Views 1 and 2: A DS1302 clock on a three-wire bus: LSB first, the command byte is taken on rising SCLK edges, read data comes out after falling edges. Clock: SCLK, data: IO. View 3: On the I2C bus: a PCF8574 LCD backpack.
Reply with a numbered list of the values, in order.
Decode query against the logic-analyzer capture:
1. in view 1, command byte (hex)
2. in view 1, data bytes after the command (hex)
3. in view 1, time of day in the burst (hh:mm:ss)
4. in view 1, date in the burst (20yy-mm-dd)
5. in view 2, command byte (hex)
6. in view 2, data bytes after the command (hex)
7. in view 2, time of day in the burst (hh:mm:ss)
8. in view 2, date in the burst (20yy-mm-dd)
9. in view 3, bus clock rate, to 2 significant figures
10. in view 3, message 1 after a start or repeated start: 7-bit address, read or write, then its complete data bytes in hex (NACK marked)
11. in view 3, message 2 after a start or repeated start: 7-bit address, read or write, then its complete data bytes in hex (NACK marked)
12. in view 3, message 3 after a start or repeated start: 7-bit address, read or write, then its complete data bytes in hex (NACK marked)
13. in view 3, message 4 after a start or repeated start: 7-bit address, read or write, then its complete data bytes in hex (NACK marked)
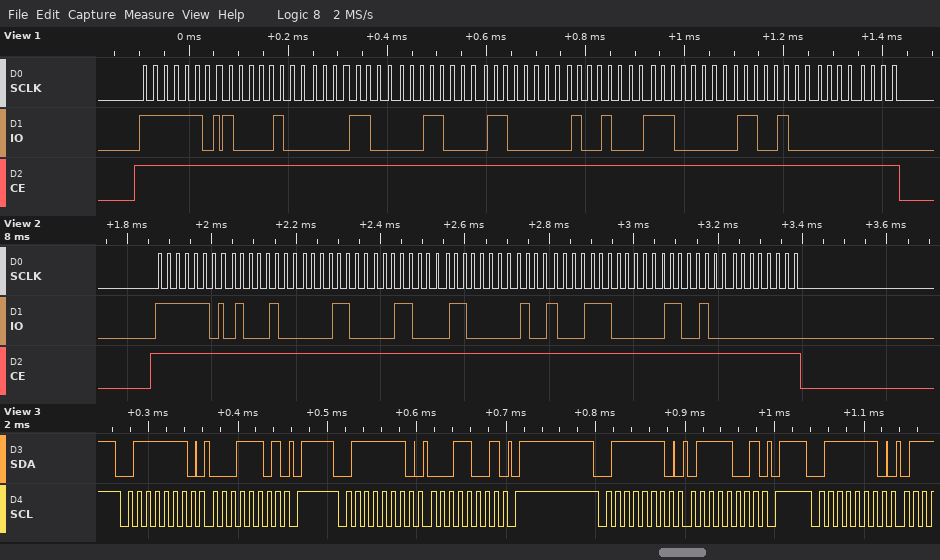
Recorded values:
1. 0xBF
2. 21 30 18 06 12 07 26 00
3. 18:30:21
4. 2026-12-06
5. 0xBF
6. 22 30 18 06 12 07 26 00
7. 18:30:22
8. 2026-12-06
9. 100 kHz
10. 0x3F write: 1D
11. 0x3F write: 19
12. 0x3F write: 79
13. 0x3F write
